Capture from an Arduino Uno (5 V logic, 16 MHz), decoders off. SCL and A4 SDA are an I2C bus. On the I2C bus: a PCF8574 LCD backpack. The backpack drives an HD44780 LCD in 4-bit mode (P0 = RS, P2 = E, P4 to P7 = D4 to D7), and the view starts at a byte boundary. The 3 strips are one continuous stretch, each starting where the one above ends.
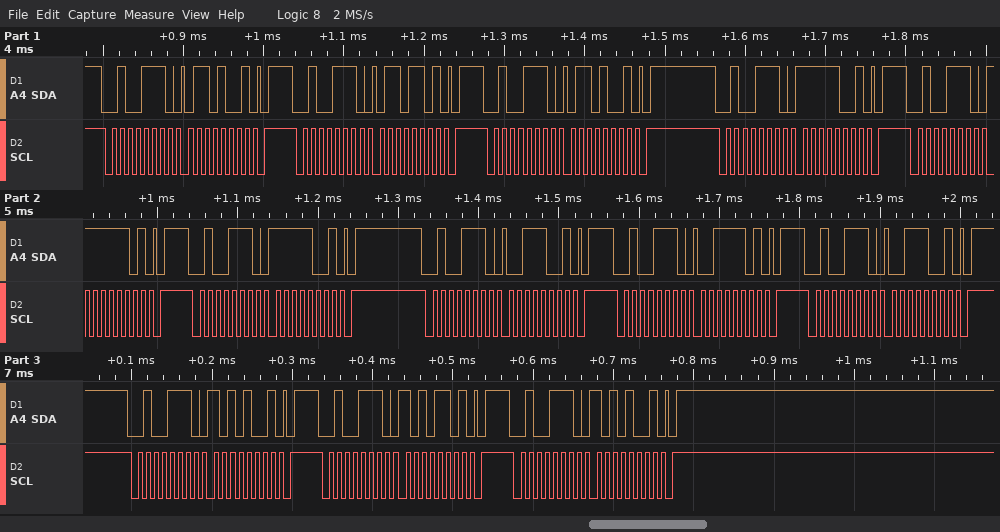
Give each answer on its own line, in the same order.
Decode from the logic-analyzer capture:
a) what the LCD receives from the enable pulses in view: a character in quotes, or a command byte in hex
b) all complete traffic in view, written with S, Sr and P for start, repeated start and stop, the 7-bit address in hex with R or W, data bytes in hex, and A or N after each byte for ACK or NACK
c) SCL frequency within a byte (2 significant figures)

'o' ':'
S 27W A 69 A P S 27W A 6D A P S 27W A 69 A P S 27W A F9 A P S 27W A FD A P S 27W A F9 A P S 27W A 39 A P S 27W A 3D A P S 27W A 39 A P S 27W A A9 A P S 27W A AD A P S 27W A A9 A P
100 kHz
